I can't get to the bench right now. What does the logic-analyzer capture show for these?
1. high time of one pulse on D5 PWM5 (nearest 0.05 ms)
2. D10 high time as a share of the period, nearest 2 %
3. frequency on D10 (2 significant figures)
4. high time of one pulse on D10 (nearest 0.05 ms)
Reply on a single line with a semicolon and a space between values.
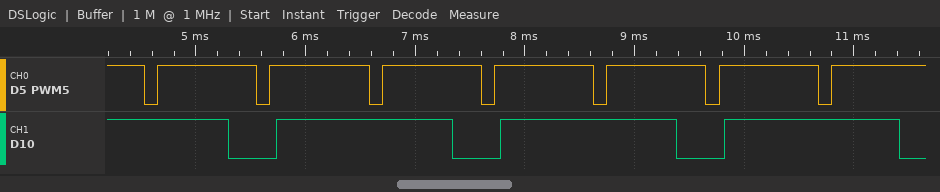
0.90 ms; 78 %; 490 Hz; 1.60 ms
